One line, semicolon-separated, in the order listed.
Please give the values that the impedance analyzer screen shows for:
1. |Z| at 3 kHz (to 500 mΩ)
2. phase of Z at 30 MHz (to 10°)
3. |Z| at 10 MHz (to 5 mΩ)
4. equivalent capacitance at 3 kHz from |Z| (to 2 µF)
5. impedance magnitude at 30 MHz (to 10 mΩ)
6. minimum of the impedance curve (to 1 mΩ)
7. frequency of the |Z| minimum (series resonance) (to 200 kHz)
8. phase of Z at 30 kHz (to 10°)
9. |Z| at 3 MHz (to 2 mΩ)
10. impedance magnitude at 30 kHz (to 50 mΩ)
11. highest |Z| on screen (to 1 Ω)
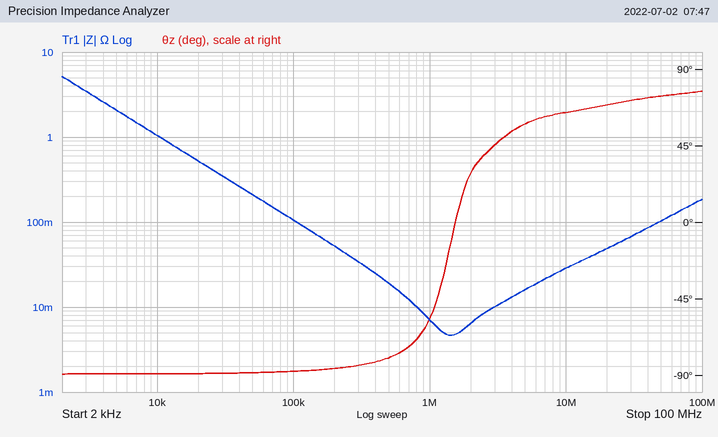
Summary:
3.5 Ω; 70°; 30 mΩ; 16 µF; 70 mΩ; 5 mΩ; 1.4 MHz; -90°; 10 mΩ; 350 mΩ; 5 Ω
